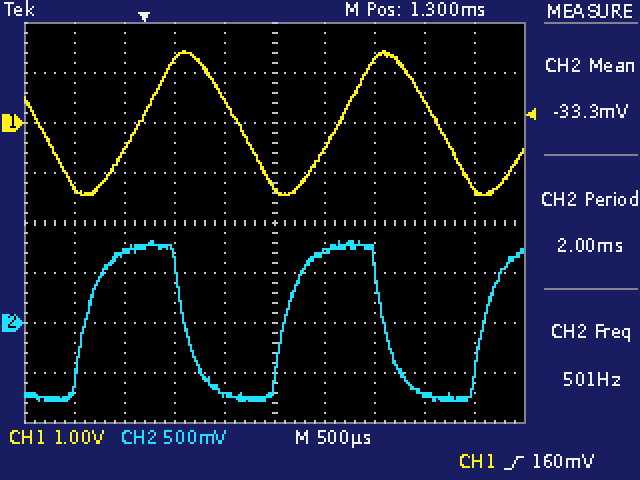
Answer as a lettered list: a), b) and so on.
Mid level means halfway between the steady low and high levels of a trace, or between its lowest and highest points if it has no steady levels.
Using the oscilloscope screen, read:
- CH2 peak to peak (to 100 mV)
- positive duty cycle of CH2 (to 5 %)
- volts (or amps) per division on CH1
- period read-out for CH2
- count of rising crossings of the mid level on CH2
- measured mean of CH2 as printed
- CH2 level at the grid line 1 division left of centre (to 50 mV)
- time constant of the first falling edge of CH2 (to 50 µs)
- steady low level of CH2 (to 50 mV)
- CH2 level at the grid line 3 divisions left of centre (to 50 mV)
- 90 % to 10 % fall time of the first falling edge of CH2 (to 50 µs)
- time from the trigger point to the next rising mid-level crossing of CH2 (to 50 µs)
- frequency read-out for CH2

a) 1.60 V
b) 50 %
c) 1 V
d) 2.00 ms
e) 3
f) -33.3 mV
g) -700 mV
h) 150 µs
i) -750 mV
j) 700 mV
k) 350 µs
l) 1.40 ms
m) 501 Hz
